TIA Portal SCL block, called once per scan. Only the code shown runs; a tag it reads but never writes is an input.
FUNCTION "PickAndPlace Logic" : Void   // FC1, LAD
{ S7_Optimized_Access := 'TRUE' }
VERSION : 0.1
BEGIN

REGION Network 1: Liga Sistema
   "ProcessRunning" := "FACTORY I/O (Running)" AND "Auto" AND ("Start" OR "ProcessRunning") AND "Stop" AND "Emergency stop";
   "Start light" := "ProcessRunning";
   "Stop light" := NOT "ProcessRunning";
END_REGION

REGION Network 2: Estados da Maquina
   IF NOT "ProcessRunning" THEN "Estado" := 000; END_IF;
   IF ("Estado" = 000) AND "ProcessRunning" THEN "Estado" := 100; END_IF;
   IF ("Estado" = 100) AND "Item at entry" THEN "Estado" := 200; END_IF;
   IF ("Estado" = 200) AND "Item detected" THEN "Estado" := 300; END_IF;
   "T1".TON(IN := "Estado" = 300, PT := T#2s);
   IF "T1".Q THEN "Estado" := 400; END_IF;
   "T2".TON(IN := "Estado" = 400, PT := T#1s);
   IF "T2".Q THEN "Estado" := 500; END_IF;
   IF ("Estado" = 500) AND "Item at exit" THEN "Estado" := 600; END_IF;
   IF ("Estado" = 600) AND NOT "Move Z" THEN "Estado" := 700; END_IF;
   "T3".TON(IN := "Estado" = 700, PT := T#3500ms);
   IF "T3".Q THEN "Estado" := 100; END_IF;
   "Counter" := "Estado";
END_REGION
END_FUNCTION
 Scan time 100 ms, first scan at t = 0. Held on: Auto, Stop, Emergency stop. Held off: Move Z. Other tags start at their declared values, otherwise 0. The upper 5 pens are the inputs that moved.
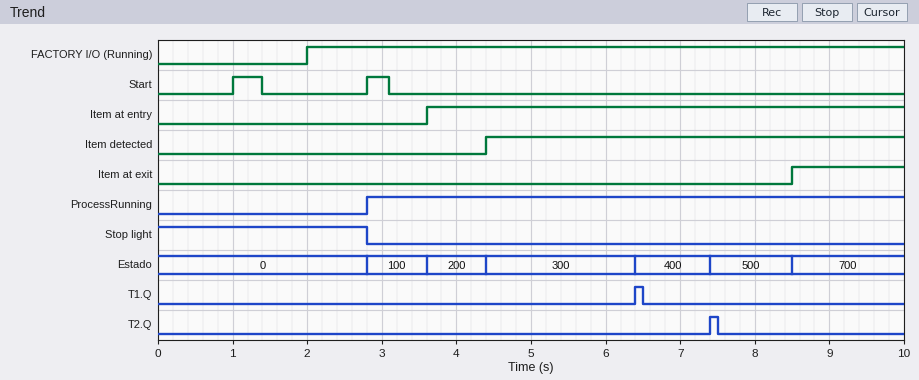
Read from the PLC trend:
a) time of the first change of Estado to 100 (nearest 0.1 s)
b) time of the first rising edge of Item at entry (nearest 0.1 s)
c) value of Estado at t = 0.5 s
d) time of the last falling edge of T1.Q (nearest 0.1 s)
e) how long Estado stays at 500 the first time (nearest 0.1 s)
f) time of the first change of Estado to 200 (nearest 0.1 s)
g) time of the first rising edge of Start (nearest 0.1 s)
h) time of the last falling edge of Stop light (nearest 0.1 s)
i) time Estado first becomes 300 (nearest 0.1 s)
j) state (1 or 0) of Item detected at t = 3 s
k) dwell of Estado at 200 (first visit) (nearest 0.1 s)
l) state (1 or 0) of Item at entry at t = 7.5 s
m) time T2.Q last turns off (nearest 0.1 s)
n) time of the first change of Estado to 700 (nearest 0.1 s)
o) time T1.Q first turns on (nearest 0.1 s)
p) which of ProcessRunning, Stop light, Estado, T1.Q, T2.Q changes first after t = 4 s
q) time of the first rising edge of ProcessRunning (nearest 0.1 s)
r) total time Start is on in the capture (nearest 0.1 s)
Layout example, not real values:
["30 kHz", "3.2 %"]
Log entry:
["2.8 s", "3.6 s", "0", "6.5 s", "1.1 s", "3.6 s", "1.0 s", "2.8 s", "4.4 s", "0", "0.8 s", "1", "7.5 s", "8.5 s", "6.4 s", "Estado", "2.8 s", "0.7 s"]
